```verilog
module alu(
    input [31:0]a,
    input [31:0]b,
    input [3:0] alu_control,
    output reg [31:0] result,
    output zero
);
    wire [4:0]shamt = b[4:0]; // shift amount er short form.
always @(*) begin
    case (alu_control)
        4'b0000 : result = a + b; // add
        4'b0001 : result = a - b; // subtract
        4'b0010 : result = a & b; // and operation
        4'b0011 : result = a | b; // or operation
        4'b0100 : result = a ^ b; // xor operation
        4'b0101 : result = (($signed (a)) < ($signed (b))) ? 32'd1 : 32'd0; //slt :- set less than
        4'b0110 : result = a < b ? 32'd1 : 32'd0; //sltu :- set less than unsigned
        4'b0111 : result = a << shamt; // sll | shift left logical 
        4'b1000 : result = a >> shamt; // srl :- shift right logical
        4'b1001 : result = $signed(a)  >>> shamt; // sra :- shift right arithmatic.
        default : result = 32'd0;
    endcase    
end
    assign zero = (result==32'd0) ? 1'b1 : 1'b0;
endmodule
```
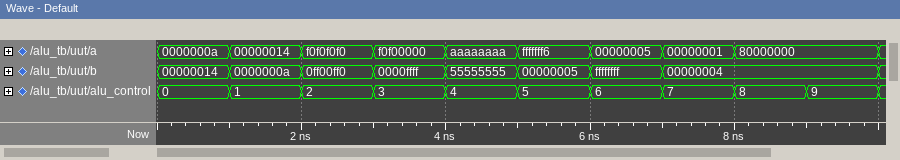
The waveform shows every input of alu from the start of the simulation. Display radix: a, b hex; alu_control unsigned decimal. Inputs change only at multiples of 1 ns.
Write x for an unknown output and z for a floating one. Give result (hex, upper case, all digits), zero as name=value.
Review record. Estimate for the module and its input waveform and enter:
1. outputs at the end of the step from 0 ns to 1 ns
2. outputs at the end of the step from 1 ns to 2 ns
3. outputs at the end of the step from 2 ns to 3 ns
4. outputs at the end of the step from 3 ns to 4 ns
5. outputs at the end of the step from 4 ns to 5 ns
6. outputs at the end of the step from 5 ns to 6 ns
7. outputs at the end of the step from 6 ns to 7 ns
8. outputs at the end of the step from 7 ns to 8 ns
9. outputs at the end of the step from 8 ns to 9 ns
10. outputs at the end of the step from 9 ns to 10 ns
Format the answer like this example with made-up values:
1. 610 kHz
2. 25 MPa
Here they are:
1. result=0000001E, zero=0
2. result=0000000A, zero=0
3. result=00F000F0, zero=0
4. result=F0F0FFFF, zero=0
5. result=FFFFFFFF, zero=0
6. result=00000001, zero=0
7. result=00000001, zero=0
8. result=00000010, zero=0
9. result=08000000, zero=0
10. result=F8000000, zero=0
